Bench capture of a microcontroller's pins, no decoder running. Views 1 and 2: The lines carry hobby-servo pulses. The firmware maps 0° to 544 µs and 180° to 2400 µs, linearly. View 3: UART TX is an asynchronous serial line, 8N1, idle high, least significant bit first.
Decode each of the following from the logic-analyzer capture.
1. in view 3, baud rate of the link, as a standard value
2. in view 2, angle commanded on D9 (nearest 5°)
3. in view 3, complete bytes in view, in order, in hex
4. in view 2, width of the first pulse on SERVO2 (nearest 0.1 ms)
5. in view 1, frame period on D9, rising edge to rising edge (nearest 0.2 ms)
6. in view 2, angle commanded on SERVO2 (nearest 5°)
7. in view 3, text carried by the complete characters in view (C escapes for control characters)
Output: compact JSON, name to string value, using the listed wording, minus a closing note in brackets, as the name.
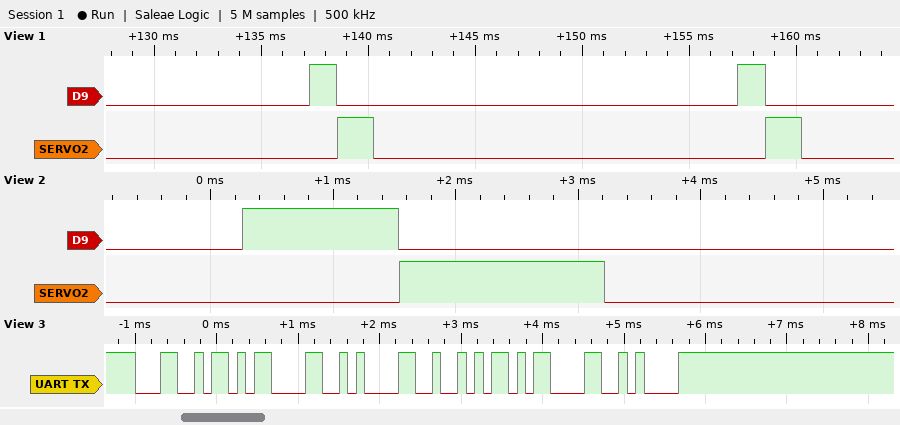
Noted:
{"in view 3, baud rate of the link, as a standard value": "9600 baud", "in view 2, angle commanded on D9": "70°", "in view 3, complete bytes in view, in order, in hex": "4C 0D 0A 52 0D 0A", "in view 2, width of the first pulse on SERVO2": "1.7 ms", "in view 1, frame period on D9, rising edge to rising edge": "20.0 ms", "in view 2, angle commanded on SERVO2": "110°", "in view 3, text carried by the complete characters in view": "\"L\\r\\nR\\r\\n\""}
